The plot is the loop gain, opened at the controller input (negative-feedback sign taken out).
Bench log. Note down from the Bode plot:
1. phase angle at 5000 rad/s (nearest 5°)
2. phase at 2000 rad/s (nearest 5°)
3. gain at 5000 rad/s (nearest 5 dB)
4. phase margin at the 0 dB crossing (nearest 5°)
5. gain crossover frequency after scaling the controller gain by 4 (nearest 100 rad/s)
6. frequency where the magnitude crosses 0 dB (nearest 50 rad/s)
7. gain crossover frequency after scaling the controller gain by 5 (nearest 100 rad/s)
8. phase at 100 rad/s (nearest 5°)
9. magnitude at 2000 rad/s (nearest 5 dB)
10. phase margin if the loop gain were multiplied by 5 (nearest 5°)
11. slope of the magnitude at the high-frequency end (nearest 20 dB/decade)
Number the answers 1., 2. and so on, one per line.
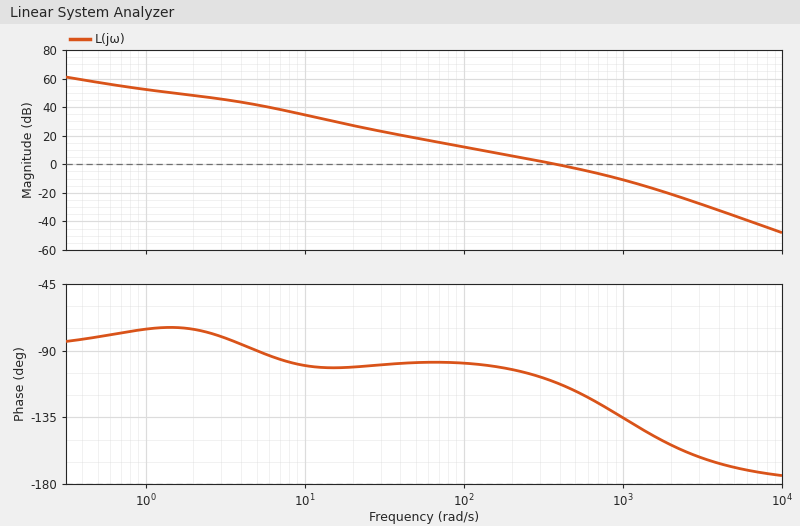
1. -170°
2. -155°
3. -35 dB
4. 70°
5. 1100 rad/s
6. 400 rad/s
7. 1300 rad/s
8. -100°
9. -20 dB
10. 40°
11. -40 dB/decade
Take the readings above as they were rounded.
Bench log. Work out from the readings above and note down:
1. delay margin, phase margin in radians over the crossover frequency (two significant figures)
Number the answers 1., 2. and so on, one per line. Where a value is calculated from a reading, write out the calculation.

1. 70 × π / 180 / 400 = 0.0031 s
